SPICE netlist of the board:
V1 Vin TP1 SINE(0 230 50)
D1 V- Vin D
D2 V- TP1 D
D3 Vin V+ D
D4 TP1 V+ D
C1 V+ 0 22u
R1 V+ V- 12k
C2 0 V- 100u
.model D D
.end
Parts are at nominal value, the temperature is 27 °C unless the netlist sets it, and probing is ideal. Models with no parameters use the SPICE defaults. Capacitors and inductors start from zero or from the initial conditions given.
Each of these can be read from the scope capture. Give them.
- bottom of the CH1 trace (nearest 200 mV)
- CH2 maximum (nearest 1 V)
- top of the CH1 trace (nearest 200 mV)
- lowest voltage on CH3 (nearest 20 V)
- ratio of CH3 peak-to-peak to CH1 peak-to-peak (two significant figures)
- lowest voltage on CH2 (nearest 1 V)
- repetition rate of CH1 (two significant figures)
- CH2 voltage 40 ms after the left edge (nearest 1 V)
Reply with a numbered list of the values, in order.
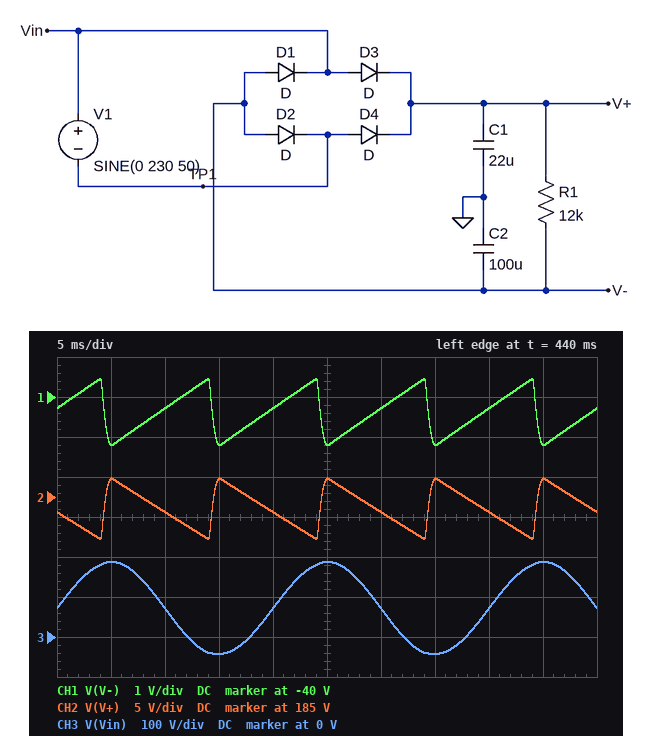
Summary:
1. -41.2 V
2. 187 V
3. -39.6 V
4. -40 V
5. 140
6. 180 V
7. 100 Hz
8. 183 V
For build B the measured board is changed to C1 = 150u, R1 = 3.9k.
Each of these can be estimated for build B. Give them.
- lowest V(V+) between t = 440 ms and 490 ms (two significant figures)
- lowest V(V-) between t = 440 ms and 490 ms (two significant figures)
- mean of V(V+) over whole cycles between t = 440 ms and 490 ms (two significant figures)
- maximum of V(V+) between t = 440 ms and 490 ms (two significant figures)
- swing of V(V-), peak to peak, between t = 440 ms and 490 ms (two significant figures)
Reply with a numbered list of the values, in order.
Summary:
1. 88 V
2. -140 V
3. 90 V
4. 91 V
5. 5.2 V
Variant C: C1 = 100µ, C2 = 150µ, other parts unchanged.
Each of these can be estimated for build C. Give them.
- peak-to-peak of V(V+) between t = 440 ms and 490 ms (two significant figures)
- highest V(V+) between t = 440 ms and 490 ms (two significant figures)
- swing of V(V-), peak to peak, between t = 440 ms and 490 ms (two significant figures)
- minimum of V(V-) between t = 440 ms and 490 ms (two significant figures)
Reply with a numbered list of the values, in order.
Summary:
1. 1.8 V
2. 140 V
3. 1.2 V
4. -91 V
